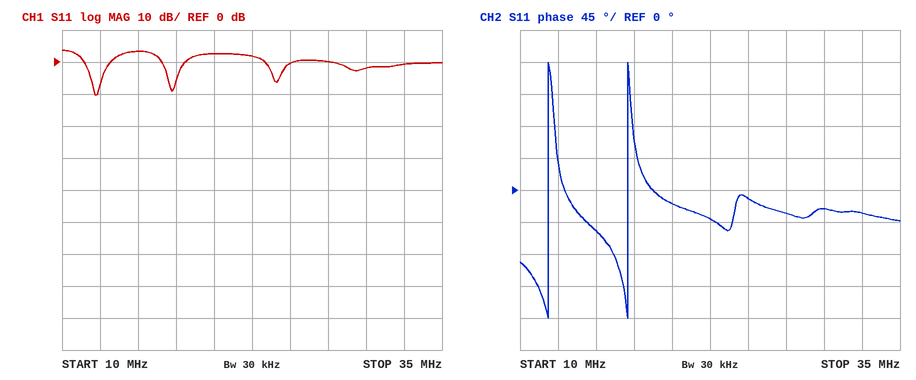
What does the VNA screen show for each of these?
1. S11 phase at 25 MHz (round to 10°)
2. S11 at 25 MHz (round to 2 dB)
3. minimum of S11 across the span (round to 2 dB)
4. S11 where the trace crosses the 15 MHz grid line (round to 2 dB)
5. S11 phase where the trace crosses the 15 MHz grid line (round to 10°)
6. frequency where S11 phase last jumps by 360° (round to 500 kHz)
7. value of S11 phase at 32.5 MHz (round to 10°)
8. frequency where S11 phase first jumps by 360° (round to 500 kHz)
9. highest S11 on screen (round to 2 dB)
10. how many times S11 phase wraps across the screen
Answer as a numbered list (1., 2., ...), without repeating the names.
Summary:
1. -10°
2. 0 dB
3. -10 dB
4. 4 dB
5. -60°
6. 17.0 MHz
7. -30°
8. 12.0 MHz
9. 4 dB
10. 2
